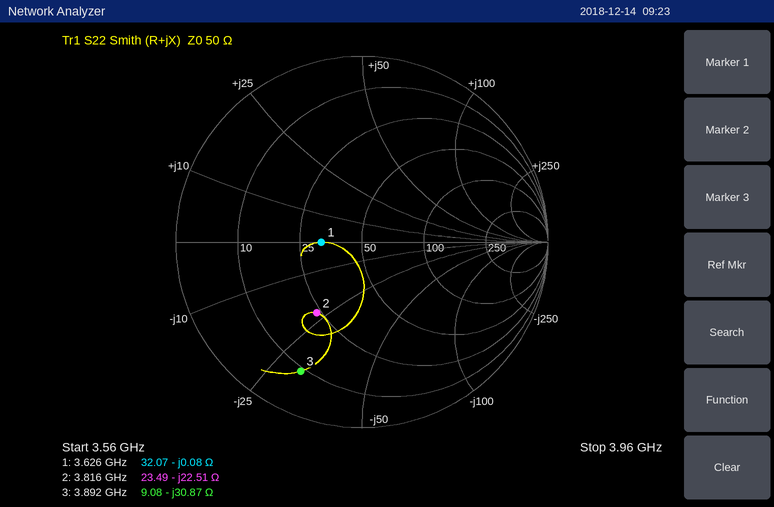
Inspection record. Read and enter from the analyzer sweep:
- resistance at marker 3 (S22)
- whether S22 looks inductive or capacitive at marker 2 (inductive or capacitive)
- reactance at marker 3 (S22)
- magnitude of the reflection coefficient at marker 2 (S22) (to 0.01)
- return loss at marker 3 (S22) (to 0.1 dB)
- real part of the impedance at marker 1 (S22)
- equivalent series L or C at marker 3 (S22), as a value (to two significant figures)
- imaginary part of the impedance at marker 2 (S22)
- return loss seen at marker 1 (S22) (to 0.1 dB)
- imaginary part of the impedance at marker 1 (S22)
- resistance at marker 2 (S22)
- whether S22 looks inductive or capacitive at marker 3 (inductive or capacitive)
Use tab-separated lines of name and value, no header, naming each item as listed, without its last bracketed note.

resistance at marker 3	9.08 Ω
whether S22 looks inductive or capacitive at marker 2	capacitive
reactance at marker 3	-30.87 Ω
magnitude of the reflection coefficient at marker 2 (S22)	0.45
return loss at marker 3 (S22)	2.3 dB
real part of the impedance at marker 1	32.07 Ω
equivalent series L or C at marker 3 (S22), as a value	1.3 pF
imaginary part of the impedance at marker 2	-22.51 Ω
return loss seen at marker 1 (S22)	13.2 dB
imaginary part of the impedance at marker 1	-0.08 Ω
resistance at marker 2	23.49 Ω
whether S22 looks inductive or capacitive at marker 3	capacitive
